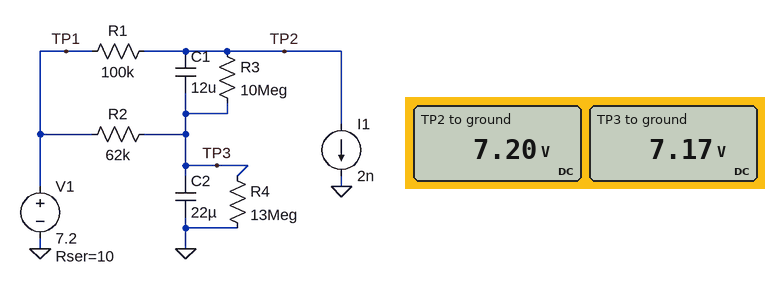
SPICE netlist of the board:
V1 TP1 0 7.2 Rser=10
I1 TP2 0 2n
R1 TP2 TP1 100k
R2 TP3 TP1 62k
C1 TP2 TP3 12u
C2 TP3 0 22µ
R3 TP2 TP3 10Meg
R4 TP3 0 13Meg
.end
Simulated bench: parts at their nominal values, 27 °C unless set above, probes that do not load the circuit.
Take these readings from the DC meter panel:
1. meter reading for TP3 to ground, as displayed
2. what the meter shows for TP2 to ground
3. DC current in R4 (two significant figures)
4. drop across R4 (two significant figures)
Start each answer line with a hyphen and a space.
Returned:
- 7.17 V
- 7.20 V
- 550 nA
- 7.2 V
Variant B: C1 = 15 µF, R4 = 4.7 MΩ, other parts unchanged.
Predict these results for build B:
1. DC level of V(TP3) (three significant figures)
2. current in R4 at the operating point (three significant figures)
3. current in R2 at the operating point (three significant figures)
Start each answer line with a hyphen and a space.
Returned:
- 7.11 V
- 1.51 µA
- 1.50 µA
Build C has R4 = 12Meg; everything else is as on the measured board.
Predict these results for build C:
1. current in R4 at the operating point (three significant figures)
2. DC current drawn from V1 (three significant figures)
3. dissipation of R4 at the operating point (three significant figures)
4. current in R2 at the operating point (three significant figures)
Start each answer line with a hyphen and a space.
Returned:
- 597 nA
- 599 nA
- 4.28 µW
- 593 nA
